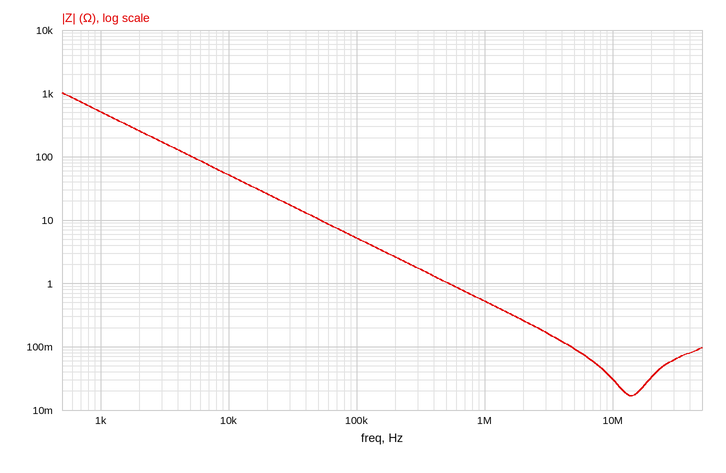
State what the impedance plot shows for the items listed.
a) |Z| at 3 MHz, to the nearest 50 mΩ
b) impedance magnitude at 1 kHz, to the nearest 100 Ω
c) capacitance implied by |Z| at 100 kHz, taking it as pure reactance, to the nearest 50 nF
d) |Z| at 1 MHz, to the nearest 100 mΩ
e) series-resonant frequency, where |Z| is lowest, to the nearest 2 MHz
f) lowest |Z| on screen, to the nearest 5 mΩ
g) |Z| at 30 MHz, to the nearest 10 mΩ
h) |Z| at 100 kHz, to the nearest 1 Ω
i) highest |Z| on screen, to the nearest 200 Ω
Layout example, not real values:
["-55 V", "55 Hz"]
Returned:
["150 mΩ", "500 Ω", "300 nF", "500 mΩ", "14 MHz", "15 mΩ", "60 mΩ", "5 Ω", "1.0 kΩ"]
